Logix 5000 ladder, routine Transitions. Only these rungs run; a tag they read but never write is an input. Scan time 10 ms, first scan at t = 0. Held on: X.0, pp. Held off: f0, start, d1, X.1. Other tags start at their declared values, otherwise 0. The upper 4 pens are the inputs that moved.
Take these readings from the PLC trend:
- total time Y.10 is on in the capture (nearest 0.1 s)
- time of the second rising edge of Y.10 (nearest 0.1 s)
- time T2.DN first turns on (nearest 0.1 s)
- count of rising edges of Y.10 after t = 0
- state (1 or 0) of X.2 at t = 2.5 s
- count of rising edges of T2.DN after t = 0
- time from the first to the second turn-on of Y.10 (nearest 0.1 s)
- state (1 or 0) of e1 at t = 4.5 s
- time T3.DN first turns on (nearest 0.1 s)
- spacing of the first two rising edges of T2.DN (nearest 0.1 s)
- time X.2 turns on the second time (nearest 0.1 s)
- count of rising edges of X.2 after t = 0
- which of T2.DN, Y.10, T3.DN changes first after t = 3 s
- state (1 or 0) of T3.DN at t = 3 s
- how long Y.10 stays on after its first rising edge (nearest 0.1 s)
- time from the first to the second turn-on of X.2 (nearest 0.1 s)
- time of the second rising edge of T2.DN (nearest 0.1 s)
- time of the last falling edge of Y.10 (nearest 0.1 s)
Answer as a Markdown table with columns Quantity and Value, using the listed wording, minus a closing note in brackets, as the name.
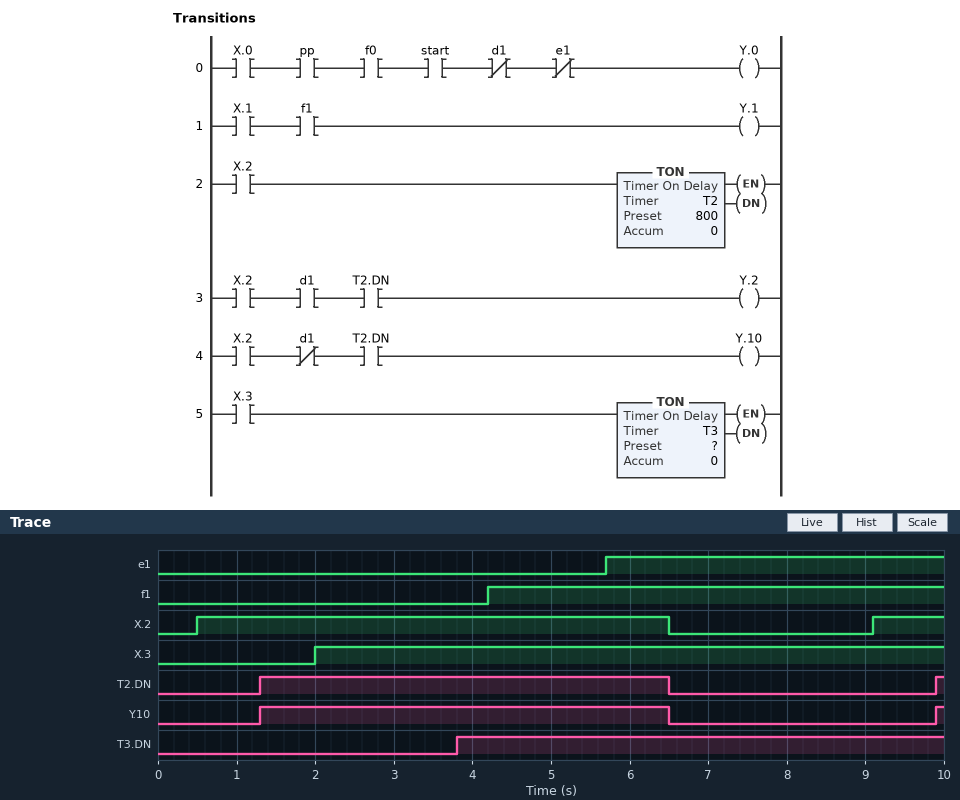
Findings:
| Quantity | Value |
|---|---|
| total time Y.10 is on in the capture | 5.3 s |
| time of the second rising edge of Y.10 | 9.9 s |
| time T2.DN first turns on | 1.3 s |
| count of rising edges of Y.10 after t = 0 | 2 |
| state (1 or 0) of X.2 at t = 2.5 s | 1 |
| count of rising edges of T2.DN after t = 0 | 2 |
| time from the first to the second turn-on of Y.10 | 8.6 s |
| state (1 or 0) of e1 at t = 4.5 s | 0 |
| time T3.DN first turns on | 3.8 s |
| spacing of the first two rising edges of T2.DN | 8.6 s |
| time X.2 turns on the second time | 9.1 s |
| count of rising edges of X.2 after t = 0 | 2 |
| which of T2.DN, Y.10, T3.DN changes first after t = 3 s | T3.DN |
| state (1 or 0) of T3.DN at t = 3 s | 0 |
| how long Y.10 stays on after its first rising edge | 5.2 s |
| time from the first to the second turn-on of X.2 | 8.6 s |
| time of the second rising edge of T2.DN | 9.9 s |
| time of the last falling edge of Y.10 | 6.5 s |
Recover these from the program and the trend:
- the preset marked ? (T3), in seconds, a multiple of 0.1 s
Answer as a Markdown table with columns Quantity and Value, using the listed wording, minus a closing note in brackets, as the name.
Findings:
| Quantity | Value |
|---|---|
| the preset marked ? (T3), in seconds, a multiple of 0.1 s | 1.8 s |
